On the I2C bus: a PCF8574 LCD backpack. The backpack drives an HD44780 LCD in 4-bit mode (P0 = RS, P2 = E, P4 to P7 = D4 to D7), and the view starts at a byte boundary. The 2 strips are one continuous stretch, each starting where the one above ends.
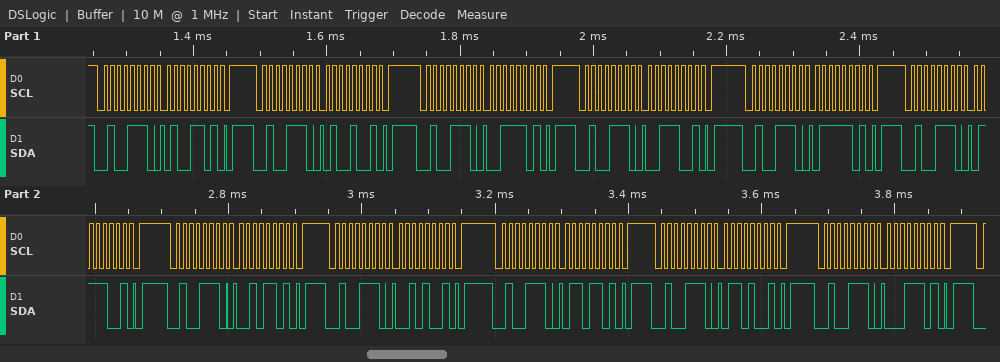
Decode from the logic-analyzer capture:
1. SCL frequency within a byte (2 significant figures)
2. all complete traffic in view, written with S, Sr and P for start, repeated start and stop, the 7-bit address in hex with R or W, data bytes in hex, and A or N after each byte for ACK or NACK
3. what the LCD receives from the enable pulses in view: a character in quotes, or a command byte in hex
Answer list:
100 kHz
S 27W A 4D A P S 27W A 49 A P S 27W A 3D A P S 27W A 39 A P S 27W A 7D A P S 27W A 79 A P S 27W A 2D A P S 27W A 29 A P S 27W A 6D A P S 27W A 69 A P S 27W A 1D A P
'C' 'r'
